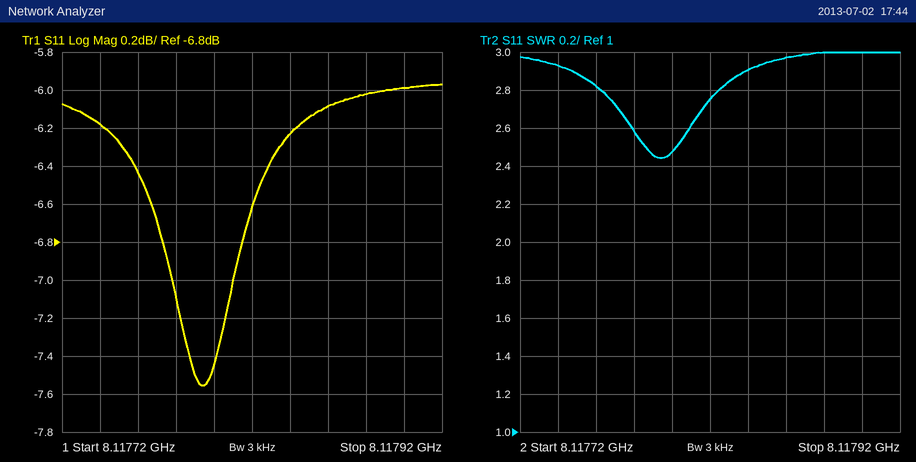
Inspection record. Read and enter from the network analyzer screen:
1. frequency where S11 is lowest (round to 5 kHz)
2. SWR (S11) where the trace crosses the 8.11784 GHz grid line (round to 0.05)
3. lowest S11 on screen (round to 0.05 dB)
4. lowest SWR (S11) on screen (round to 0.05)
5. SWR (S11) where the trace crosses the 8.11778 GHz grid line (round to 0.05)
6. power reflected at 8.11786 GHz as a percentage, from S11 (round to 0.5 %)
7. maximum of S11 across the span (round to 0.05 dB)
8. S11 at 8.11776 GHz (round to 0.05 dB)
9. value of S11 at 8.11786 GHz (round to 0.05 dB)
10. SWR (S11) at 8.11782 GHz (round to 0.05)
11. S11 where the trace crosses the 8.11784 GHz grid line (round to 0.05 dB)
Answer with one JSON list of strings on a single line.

["8.117795 GHz", "2.90", "-7.55 dB", "2.45", "2.60", "24.5 %", "-5.95 dB", "-6.45 dB", "-6.10 dB", "2.75", "-6.25 dB"]
